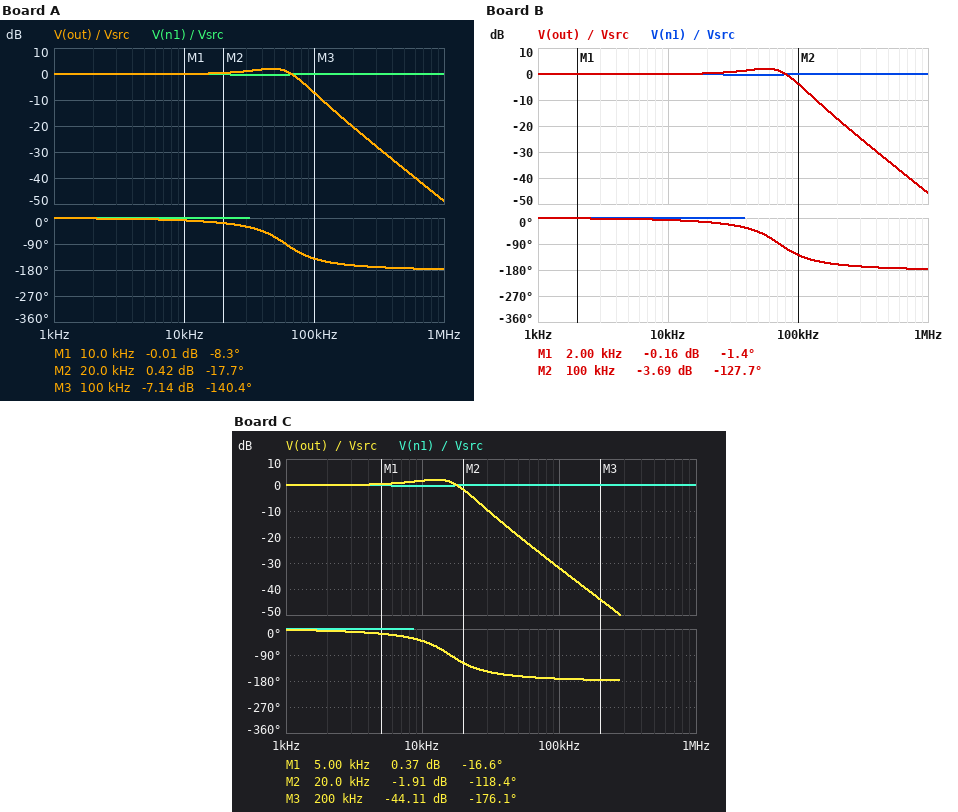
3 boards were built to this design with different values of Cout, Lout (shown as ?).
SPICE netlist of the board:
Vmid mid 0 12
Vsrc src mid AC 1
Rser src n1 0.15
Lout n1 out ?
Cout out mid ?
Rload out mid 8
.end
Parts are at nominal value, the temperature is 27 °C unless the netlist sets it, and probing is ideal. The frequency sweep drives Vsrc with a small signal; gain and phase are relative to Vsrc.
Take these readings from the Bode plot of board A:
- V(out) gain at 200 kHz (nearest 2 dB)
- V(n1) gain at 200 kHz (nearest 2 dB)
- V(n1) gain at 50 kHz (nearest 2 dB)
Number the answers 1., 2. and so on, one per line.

1. -20 dB
2. 0 dB
3. 0 dB
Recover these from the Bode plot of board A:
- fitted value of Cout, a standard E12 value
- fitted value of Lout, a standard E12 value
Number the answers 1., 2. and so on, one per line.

1. 390 nF
2. 18 µH
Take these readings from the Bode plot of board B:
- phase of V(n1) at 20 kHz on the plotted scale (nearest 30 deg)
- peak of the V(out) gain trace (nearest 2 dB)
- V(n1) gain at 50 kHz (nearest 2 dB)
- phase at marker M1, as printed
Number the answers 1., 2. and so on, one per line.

1. 0 deg
2. 2 dB
3. 0 dB
4. -1.4 deg
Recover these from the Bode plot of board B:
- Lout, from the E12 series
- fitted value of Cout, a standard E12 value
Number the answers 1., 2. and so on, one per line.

1. 15 µH
2. 330 nF
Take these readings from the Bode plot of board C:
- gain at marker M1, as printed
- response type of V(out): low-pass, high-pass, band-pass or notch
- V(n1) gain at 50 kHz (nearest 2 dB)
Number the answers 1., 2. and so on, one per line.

1. 0.37 dB
2. low-pass
3. 0 dB
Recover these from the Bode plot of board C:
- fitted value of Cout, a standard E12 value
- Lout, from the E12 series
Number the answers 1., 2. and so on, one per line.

1. 1.5 µF
2. 68 µH
